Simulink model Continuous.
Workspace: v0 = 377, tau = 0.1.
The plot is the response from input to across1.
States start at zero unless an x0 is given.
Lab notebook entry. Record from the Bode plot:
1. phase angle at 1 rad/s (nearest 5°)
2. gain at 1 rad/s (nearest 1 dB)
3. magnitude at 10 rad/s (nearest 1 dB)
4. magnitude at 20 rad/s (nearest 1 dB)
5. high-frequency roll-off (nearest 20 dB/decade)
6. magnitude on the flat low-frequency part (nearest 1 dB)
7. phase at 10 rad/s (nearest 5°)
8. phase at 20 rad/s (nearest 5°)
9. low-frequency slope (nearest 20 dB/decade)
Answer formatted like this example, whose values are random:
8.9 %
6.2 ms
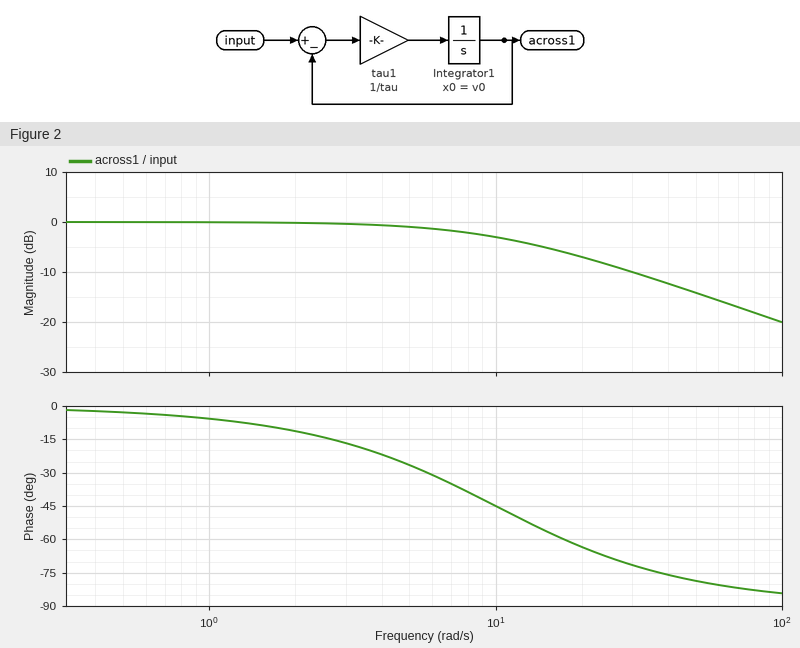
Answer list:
-5°
0 dB
-3 dB
-7 dB
-20 dB/decade
0 dB
-45°
-65°
0 dB/decade
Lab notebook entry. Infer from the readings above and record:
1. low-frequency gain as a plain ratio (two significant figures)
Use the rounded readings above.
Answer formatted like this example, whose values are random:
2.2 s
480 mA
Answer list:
1.0
